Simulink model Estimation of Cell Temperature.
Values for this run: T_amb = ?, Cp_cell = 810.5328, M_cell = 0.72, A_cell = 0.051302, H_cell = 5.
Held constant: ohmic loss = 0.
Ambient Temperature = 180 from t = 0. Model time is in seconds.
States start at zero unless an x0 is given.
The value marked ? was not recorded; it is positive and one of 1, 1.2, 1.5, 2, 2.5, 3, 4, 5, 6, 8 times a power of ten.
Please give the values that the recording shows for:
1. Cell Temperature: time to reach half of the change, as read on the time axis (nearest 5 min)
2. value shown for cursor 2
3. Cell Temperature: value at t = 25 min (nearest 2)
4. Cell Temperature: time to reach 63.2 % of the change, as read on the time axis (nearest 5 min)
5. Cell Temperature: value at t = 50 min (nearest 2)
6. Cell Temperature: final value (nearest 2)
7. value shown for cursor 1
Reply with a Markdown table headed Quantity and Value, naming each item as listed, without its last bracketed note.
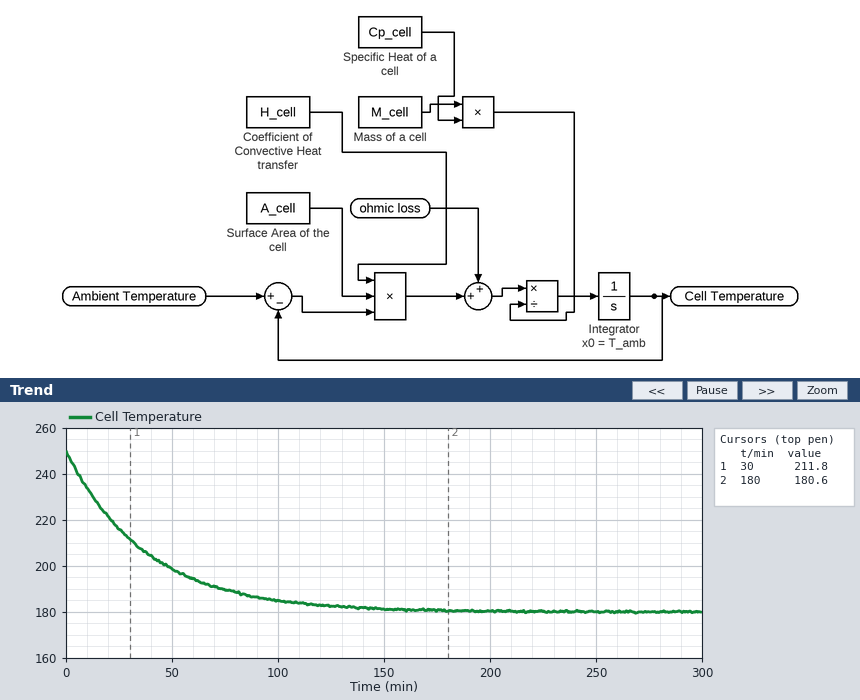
| Quantity | Value |
|---|---|
| Cell Temperature: time to reach half of the change, as read on the time axis | 25 min |
| value shown for cursor 2 | 180.6 |
| Cell Temperature: value at t = 25 min | 216 |
| Cell Temperature: time to reach 63.2 % of the change, as read on the time axis | 40 min |
| Cell Temperature: value at t = 50 min | 198 |
| Cell Temperature: final value | 180 |
| value shown for cursor 1 | 211.8 |
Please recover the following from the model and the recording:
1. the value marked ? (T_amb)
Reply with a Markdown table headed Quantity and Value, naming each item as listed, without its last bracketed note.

| Quantity | Value |
|---|---|
| the value marked ? | 250 |
